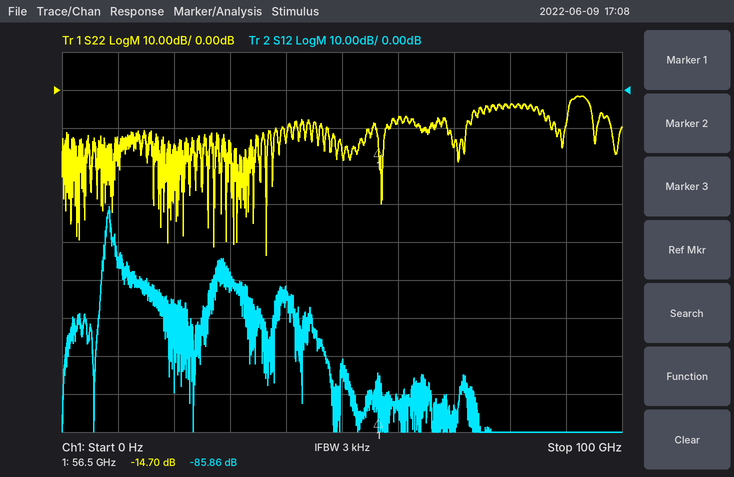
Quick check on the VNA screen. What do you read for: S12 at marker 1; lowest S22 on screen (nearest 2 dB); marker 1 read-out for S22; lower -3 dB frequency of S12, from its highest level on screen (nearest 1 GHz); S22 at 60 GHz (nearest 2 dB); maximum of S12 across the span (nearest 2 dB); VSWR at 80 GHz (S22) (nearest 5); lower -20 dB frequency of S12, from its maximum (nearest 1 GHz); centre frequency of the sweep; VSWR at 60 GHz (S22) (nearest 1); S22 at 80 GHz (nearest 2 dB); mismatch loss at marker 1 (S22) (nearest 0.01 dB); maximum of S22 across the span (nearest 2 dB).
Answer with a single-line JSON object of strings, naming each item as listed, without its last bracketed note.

{"S12 at marker 1": "-85.86 dB", "lowest S22 on screen": "-44 dB", "marker 1 read-out for S22": "-14.70 dB", "lower -3 dB frequency of S12, from its highest level on screen": "8 GHz", "S22 at 60 GHz": "-8 dB", "maximum of S12 across the span": "-30 dB", "VSWR at 80 GHz (S22)": "5", "lower -20 dB frequency of S12, from its maximum": "7 GHz", "centre frequency of the sweep": "50 GHz", "VSWR at 60 GHz (S22)": "2", "S22 at 80 GHz": "-4 dB", "mismatch loss at marker 1 (S22)": "0.15 dB", "maximum of S22 across the span": "-2 dB"}
